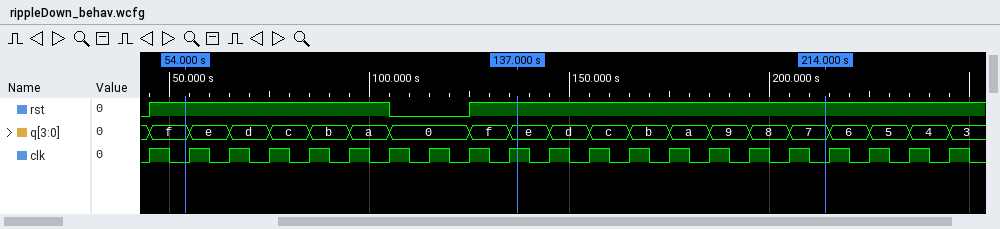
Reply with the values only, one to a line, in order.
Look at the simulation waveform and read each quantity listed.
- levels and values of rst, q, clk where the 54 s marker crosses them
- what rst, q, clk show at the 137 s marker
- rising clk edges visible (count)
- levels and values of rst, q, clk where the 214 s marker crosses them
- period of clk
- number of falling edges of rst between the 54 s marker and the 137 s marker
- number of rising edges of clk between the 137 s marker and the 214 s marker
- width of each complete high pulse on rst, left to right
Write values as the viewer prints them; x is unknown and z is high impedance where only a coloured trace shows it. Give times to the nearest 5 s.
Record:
rst=1, q=f, clk=0
rst=1, q=e, clk=1
21
rst=1, q=7, clk=0
10 s
1
7
60 s
